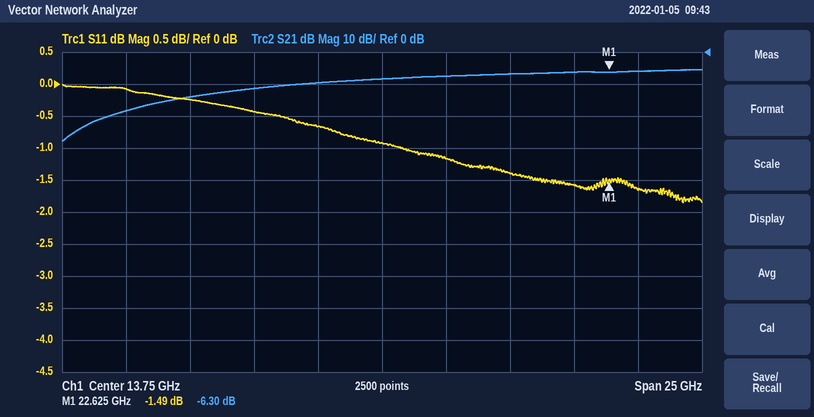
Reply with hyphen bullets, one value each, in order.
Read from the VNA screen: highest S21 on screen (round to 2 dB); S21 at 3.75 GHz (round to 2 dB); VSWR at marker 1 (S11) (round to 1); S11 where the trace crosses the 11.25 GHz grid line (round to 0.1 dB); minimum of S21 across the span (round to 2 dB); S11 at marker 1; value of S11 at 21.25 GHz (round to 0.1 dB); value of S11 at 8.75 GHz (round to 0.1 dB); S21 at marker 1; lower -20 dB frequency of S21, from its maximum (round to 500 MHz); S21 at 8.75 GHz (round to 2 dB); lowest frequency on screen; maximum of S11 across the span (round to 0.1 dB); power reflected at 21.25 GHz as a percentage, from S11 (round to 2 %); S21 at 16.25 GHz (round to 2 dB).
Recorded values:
- -6 dB
- -18 dB
- 12
- -0.7 dB
- -28 dB
- -1.49 dB
- -1.6 dB
- -0.4 dB
- -6.30 dB
- 1.5 GHz
- -12 dB
- 1.25 GHz
- 0.0 dB
- 70 %
- -8 dB
